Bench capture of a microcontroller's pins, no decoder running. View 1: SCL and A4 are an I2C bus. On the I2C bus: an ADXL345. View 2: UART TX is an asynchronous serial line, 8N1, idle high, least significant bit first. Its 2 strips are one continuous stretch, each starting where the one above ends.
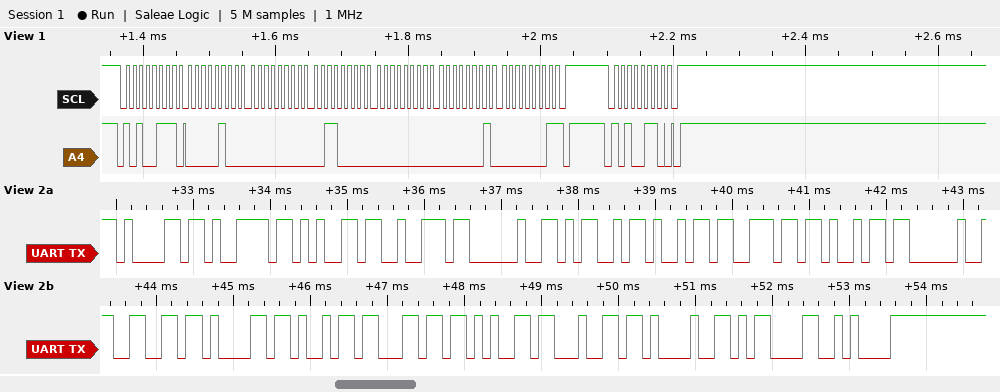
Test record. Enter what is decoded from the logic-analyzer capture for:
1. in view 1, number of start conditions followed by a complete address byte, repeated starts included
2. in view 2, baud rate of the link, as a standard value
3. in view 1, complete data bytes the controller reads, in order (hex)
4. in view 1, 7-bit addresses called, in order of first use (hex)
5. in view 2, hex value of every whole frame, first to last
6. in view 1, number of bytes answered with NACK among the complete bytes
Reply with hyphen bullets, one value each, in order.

- 2
- 9600 baud
- 04 00 30 00 01 01
- 0x53
- 0x61 0x79 0x65 0x72 0x20 0x4D 0x69 0x6E 0x69 0x20 0x66 0x61 0x69 0x6C 0x65 0x64 0x21 0x0D 0x0A
- 1
